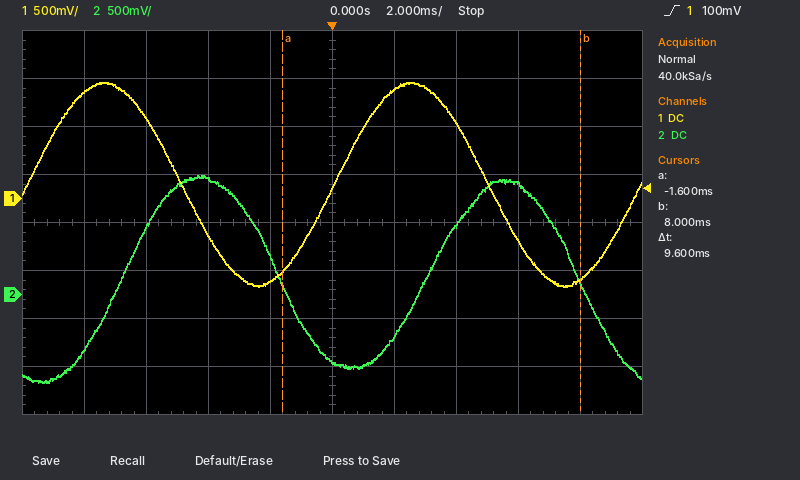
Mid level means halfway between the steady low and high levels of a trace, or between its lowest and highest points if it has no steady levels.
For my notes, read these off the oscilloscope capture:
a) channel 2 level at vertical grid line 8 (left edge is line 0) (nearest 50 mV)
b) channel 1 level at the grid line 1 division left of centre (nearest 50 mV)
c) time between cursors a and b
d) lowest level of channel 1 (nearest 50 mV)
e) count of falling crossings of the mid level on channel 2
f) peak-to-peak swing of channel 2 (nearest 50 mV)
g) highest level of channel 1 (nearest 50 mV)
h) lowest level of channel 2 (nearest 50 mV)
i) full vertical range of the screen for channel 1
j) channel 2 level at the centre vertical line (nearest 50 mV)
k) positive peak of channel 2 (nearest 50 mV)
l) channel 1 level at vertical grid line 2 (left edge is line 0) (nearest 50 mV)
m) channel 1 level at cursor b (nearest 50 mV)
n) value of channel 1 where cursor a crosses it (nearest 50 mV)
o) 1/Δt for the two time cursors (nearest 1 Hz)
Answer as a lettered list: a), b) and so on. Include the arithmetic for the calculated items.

a) 1.15 V
b) -850 mV
c) 9.6 ms
d) -900 mV
e) 2
f) 1.25 V − (-900 mV) = 2.15 V
g) 1.20 V
h) -900 mV
i) 4 V
j) -700 mV
k) 1.25 V
l) 850 mV
m) -850 mV
n) -750 mV
o) 1 / 9.6 ms ≈ 104 Hz
